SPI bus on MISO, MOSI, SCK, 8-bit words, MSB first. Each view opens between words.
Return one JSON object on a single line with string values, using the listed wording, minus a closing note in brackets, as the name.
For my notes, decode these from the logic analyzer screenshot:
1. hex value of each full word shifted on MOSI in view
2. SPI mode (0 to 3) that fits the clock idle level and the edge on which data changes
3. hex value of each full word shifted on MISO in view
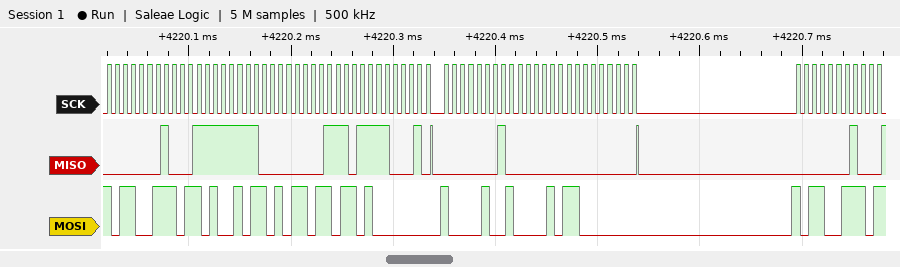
{"hex value of each full word shifted on MOSI in view": "B3, B4, B5, B6, 80, 84, 85, 80, B3", "SPI mode (0 to 3) that fits the clock idle level and the edge on which data changes": "0", "hex value of each full word shifted on MISO in view": "01, 1F, E0, 1D, E2, 01, 00, 00, 01"}
